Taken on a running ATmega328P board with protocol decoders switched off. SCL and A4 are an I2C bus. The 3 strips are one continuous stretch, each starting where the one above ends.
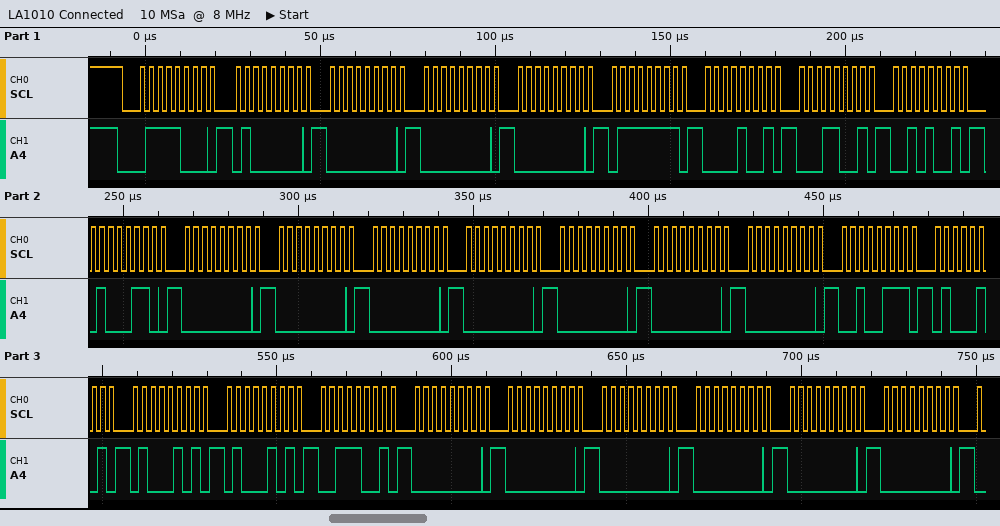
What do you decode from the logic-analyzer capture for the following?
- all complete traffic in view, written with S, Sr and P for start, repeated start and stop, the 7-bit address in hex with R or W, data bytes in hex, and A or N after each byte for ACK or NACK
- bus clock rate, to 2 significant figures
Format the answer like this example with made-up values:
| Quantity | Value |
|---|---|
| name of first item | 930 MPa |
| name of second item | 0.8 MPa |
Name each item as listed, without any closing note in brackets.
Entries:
| Quantity | Value |
|---|---|
| all complete traffic in view, written with S, Sr and P for start, repeated start and stop, the 7-bit address in hex with R or W, data bytes in hex, and A or N after each byte for ACK or NACK | S 3CW A 40 A 00 A 00 A 00 A 7F A 09 A 19 A 29 A 46 A 00 A 00 A 00 A 00 A 00 A 00 A 00 A 27 A 45 A 45 A 45 A 39 A 00 A 00 A 00 A 00 A 00 A 00 A |
| bus clock rate, to 2 significant figures | 400 kHz |
